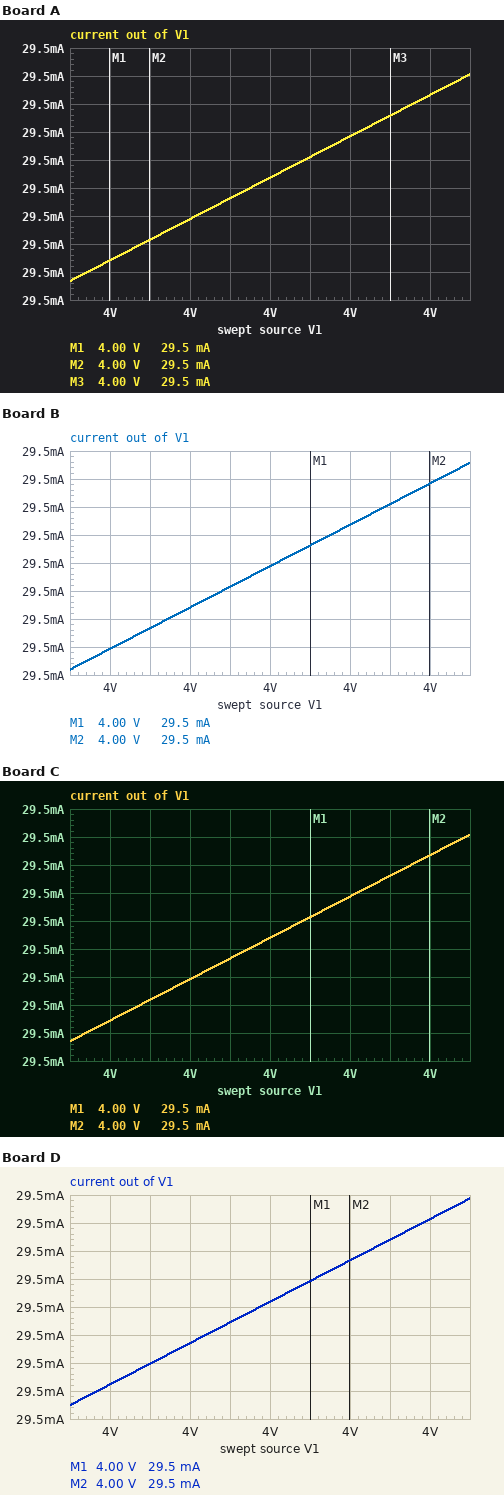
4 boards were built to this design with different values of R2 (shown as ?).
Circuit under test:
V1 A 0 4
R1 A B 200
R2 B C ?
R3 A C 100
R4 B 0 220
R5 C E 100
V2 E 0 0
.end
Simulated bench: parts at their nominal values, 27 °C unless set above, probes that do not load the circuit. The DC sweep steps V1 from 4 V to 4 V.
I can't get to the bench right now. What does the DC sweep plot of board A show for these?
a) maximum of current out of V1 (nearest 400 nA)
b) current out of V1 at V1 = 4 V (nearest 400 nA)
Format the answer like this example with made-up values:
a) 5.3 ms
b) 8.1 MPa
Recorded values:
a) 29.5340 mA
b) 29.5312 mA
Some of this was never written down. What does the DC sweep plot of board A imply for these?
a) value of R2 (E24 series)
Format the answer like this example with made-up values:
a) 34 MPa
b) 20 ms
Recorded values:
a) 620 Ω
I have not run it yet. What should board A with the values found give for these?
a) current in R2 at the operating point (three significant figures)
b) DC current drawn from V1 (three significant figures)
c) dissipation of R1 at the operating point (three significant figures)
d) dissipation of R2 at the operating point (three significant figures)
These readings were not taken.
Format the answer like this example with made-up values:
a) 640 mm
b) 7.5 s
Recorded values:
a) 123 µA
b) 29.5 mA
c) 18.4 mW
d) 9.37 µW
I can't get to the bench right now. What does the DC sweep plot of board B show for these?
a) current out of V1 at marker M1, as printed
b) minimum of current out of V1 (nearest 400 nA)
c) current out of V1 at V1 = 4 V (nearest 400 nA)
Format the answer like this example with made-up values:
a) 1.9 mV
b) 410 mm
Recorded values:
a) 29.5 mA
b) 29.5244 mA
c) 29.5288 mA
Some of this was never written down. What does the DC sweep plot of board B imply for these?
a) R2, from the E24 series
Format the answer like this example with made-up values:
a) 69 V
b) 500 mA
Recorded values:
a) 130 Ω
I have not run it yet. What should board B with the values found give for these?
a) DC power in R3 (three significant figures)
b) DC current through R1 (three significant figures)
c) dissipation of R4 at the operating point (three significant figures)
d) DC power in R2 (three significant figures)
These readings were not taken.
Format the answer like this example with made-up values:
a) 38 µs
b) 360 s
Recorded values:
a) 39.3 mW
b) 9.70 mA
c) 19.3 mW
d) 14.5 µW
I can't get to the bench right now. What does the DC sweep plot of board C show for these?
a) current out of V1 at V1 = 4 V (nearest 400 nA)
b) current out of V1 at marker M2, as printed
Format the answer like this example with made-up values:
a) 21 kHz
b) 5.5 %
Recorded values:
a) 29.5244 mA
b) 29.5 mA
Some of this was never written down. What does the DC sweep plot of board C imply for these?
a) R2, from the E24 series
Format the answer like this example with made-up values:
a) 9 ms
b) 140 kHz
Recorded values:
a) 300 Ω
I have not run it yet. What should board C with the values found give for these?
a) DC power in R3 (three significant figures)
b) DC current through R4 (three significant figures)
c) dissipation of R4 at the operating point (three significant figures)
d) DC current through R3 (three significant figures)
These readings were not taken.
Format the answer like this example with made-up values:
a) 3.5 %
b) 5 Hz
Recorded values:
a) 39.6 mW
b) 9.42 mA
c) 19.5 mW
d) 19.9 mA
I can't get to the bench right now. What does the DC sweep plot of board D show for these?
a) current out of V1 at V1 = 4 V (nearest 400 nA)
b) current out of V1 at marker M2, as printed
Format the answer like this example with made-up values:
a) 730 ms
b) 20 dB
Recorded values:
a) 29.5280 mA
b) 29.5 mA
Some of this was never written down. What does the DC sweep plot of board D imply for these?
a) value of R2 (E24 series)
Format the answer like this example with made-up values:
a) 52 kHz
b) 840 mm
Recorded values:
a) 110 Ω
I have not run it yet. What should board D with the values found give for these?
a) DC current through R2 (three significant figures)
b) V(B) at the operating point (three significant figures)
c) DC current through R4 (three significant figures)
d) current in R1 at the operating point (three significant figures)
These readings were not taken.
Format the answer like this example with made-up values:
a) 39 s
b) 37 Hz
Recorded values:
a) 360 µA
b) 2.06 V
c) 9.35 mA
d) 9.71 mA
